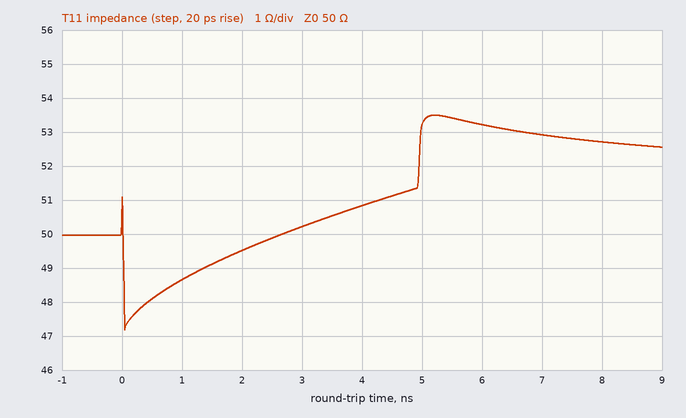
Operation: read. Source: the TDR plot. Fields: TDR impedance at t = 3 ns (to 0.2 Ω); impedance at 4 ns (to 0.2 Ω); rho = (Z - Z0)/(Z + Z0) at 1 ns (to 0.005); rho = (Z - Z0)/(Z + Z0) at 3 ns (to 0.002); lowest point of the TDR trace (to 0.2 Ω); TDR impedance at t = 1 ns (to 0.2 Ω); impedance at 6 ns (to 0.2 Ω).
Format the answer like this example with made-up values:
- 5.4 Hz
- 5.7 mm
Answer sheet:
- 50.2 Ω
- 50.8 Ω
- -0.015
- +0.002
- 47.2 Ω
- 48.6 Ω
- 53.2 Ω
